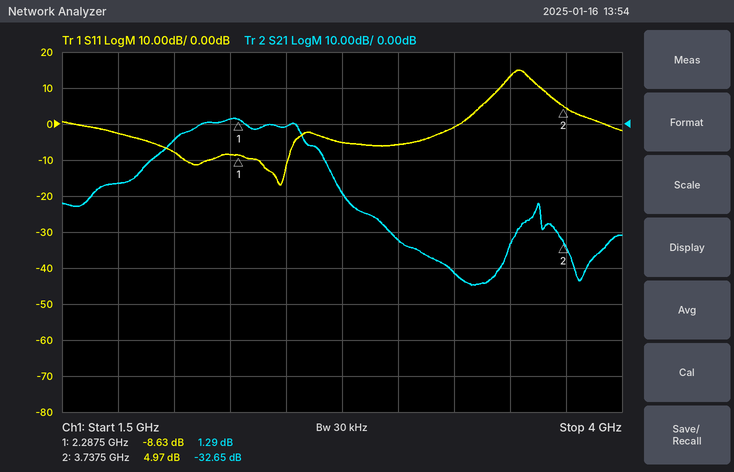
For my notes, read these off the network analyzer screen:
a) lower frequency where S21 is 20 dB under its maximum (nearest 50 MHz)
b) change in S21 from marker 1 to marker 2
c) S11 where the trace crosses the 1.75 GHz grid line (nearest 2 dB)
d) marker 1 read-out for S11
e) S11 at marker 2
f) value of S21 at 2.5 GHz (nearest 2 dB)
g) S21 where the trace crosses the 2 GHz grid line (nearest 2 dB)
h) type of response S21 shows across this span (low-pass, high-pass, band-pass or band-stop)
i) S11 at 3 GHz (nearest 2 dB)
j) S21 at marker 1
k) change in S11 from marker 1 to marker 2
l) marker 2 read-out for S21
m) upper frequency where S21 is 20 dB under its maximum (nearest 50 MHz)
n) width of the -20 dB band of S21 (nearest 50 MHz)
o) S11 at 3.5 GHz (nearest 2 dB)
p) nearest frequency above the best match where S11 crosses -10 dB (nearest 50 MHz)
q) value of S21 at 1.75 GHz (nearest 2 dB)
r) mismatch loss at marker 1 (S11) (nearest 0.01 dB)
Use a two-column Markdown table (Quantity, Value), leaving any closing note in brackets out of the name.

| Quantity | Value |
|---|---|
| lower frequency where S21 is 20 dB under its maximum | 1.65 GHz |
| change in S21 from marker 1 to marker 2 | -33.94 dB |
| S11 where the trace crosses the 1.75 GHz grid line | -2 dB |
| marker 1 read-out for S11 | -8.63 dB |
| S11 at marker 2 | 4.97 dB |
| value of S21 at 2.5 GHz | 0 dB |
| S21 where the trace crosses the 2 GHz grid line | -4 dB |
| type of response S21 shows across this span | band-pass |
| S11 at 3 GHz | -6 dB |
| S21 at marker 1 | 1.29 dB |
| change in S11 from marker 1 to marker 2 | 13.60 dB |
| marker 2 read-out for S21 | -32.65 dB |
| upper frequency where S21 is 20 dB under its maximum | 2.75 GHz |
| width of the -20 dB band of S21 | 1.10 GHz |
| S11 at 3.5 GHz | 14 dB |
| nearest frequency above the best match where S11 crosses -10 dB | 2.50 GHz |
| value of S21 at 1.75 GHz | -16 dB |
| mismatch loss at marker 1 (S11) | 0.64 dB |
